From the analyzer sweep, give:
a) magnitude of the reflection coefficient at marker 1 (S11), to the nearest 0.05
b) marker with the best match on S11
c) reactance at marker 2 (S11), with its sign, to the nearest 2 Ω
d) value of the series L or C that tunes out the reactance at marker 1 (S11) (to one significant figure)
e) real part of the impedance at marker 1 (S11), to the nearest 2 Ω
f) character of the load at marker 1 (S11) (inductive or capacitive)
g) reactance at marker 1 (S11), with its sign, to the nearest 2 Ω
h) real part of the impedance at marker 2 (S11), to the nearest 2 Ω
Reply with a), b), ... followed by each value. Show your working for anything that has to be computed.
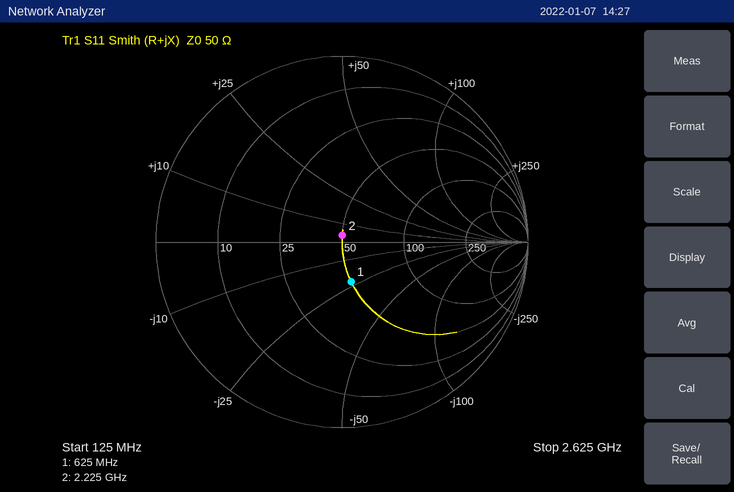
a) 0.20
b) marker 2
c) +4 Ω
d) L = 22 Ω/(2π × 625 MHz) ≈ 6 nH
e) 50 Ω
f) capacitive
g) -22 Ω
h) 50 Ω
